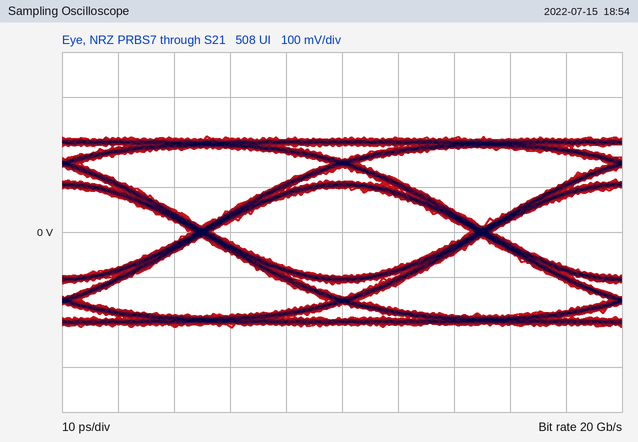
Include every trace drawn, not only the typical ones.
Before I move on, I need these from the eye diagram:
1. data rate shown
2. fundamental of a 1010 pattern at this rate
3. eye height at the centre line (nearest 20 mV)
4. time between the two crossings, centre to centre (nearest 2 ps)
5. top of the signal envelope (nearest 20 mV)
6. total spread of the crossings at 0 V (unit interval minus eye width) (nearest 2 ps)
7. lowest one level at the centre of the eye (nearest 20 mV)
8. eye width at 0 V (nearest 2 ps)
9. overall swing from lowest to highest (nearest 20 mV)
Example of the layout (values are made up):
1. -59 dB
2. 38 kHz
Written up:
1. 20 Gb/s
2. 10 GHz
3. 200 mV
4. 50 ps
5. 220 mV
6. 4 ps
7. 100 mV
8. 46 ps
9. 420 mV
